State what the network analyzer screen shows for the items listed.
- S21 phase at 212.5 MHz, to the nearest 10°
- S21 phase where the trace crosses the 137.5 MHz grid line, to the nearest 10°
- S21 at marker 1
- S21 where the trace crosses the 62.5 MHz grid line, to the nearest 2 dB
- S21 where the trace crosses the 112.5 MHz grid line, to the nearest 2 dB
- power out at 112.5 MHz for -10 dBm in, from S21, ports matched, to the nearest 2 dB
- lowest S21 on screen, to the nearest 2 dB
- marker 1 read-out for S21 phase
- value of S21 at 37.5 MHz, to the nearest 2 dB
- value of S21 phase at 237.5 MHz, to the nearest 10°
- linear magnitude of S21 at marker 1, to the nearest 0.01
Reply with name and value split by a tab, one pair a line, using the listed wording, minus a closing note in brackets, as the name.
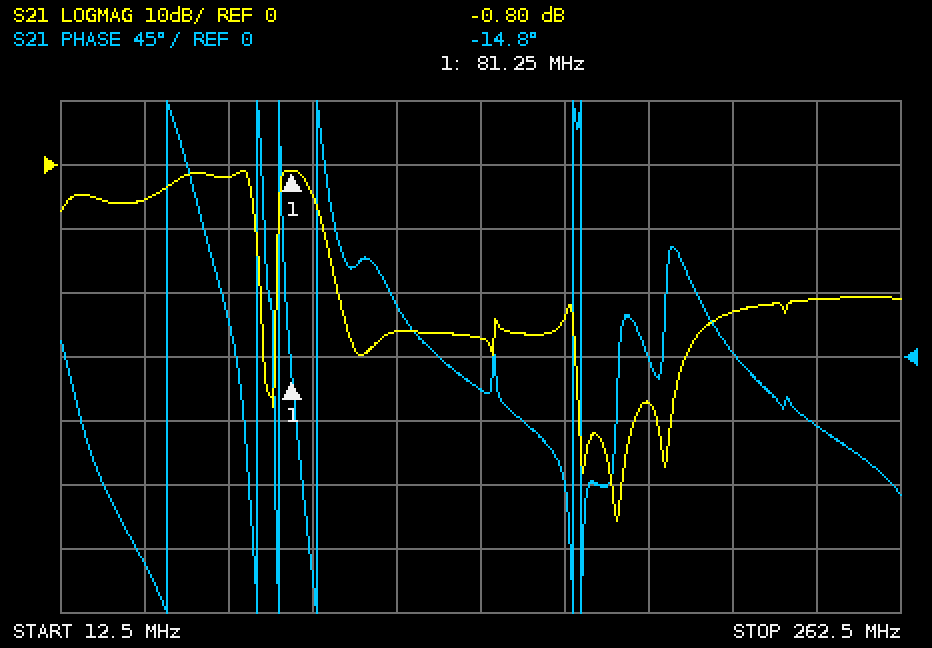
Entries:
S21 phase at 212.5 MHz, to the nearest 10°	0°
S21 phase where the trace crosses the 137.5 MHz grid line, to the nearest 10°	-20°
S21 at marker 1	-0.80 dB
S21 where the trace crosses the 62.5 MHz grid line, to the nearest 2 dB	-2 dB
S21 where the trace crosses the 112.5 MHz grid line, to the nearest 2 dB	-26 dB
power out at 112.5 MHz for -10 dBm in, from S21, ports matched, to the nearest 2 dB	-36 dBm
lowest S21 on screen, to the nearest 2 dB	-56 dB
marker 1 read-out for S21 phase	-14.8°
value of S21 at 37.5 MHz, to the nearest 2 dB	-6 dB
value of S21 phase at 237.5 MHz, to the nearest 10°	-50°
linear magnitude of S21 at marker 1, to the nearest 0.01	0.91
